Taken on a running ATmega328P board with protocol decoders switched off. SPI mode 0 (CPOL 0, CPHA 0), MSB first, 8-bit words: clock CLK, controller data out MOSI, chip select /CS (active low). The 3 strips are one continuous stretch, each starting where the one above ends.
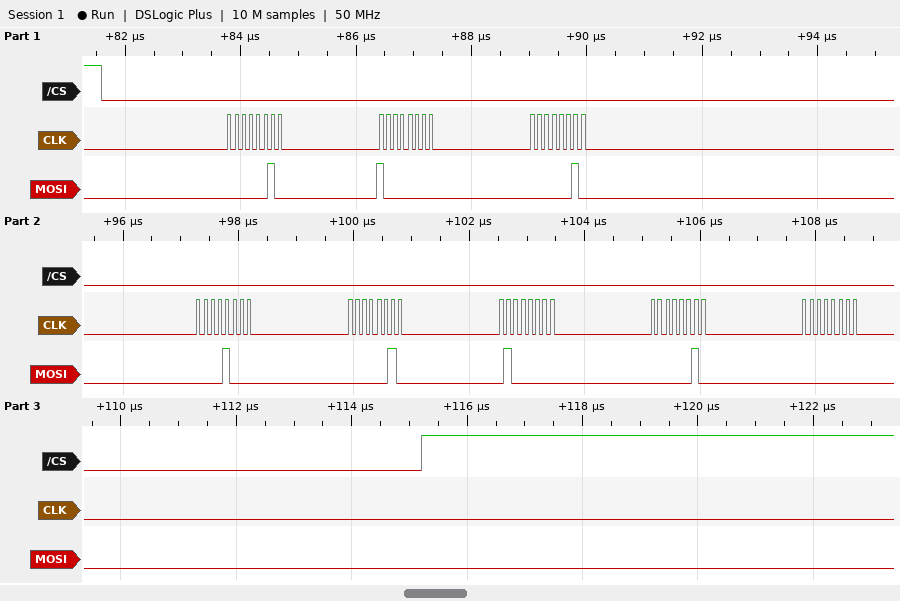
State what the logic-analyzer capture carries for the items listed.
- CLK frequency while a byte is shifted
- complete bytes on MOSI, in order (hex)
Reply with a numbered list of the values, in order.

1. 8 MHz
2. 02 80 02 08 02 40 02 00
